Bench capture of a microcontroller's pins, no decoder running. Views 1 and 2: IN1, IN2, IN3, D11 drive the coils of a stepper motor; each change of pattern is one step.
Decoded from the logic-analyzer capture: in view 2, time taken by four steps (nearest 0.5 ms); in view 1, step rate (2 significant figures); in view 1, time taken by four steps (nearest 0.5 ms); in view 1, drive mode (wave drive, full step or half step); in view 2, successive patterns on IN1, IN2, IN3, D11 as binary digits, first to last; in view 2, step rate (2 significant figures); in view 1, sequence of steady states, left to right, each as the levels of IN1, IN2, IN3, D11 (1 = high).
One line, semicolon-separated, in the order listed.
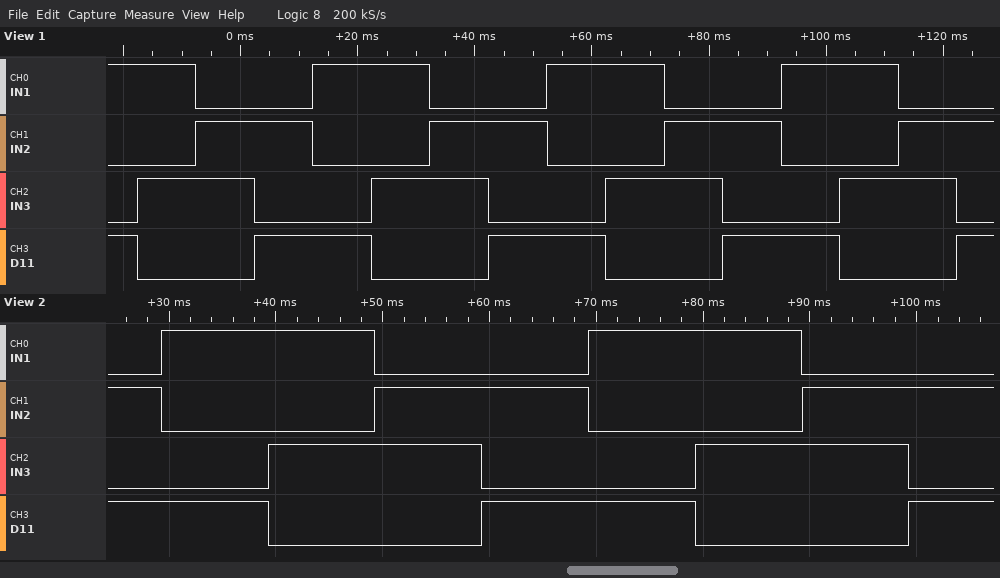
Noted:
40.0 ms; 100 steps/s; 40.0 ms; full step; 0101 1001 1010 0110 0101 1001 1010 0110 0101; 100 steps/s; 1001 1010 0110 0101 1001 1010 0110 0101 1001 1010 0110 0101 1001 1010 0110 0101
